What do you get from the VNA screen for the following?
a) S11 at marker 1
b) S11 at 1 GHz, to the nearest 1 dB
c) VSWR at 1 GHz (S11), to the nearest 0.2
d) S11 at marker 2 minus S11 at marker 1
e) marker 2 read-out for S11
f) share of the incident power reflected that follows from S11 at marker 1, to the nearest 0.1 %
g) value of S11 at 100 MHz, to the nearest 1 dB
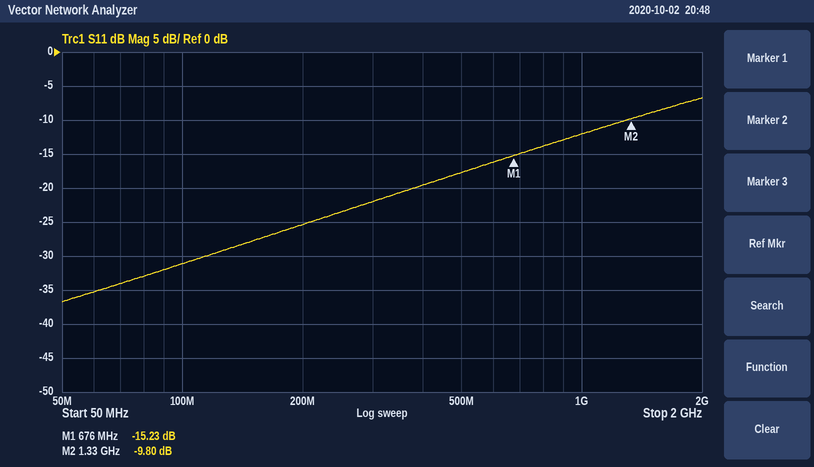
-15.23 dB
-12 dB
1.6
5.43 dB
-9.80 dB
3.0 %
-31 dB
